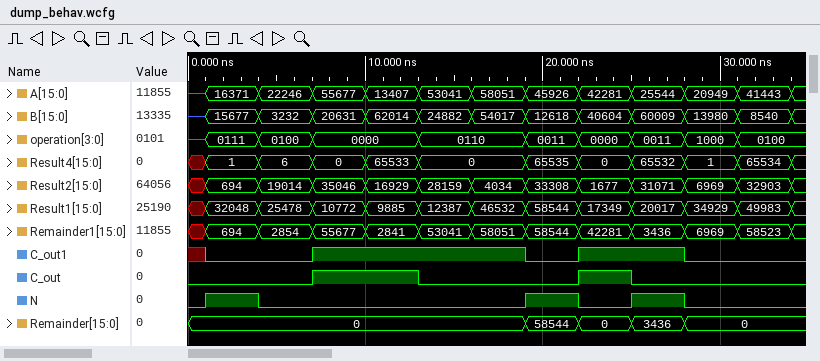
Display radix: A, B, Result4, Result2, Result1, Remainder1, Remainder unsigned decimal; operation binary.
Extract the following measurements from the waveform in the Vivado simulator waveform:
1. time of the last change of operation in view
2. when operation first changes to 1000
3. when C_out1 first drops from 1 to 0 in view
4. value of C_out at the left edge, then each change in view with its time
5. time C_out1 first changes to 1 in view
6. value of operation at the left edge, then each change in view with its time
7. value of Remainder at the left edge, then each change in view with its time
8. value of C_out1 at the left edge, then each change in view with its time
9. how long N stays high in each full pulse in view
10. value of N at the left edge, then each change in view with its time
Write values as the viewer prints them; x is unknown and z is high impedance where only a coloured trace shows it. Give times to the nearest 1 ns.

31 ns
28 ns
19 ns
0, 1 at 7 ns, 0 at 13 ns, 1 at 22 ns, 0 at 25 ns
7 ns
z, 0111 at 1 ns, 0100 at 4 ns, 0000 at 7 ns, 0110 at 13 ns, 0011 at 19 ns, 0000 at 22 ns, 0011 at 25 ns, 1000 at 28 ns, 0100 at 31 ns
0, 58544 at 19 ns, 0 at 22 ns, 3436 at 25 ns, 0 at 28 ns
x, 0 at 1 ns, 1 at 7 ns, 0 at 19 ns, 1 at 22 ns, 0 at 28 ns
3 ns, 3 ns, 3 ns
0, 1 at 1 ns, 0 at 4 ns, 1 at 19 ns, 0 at 22 ns, 1 at 25 ns, 0 at 28 ns
